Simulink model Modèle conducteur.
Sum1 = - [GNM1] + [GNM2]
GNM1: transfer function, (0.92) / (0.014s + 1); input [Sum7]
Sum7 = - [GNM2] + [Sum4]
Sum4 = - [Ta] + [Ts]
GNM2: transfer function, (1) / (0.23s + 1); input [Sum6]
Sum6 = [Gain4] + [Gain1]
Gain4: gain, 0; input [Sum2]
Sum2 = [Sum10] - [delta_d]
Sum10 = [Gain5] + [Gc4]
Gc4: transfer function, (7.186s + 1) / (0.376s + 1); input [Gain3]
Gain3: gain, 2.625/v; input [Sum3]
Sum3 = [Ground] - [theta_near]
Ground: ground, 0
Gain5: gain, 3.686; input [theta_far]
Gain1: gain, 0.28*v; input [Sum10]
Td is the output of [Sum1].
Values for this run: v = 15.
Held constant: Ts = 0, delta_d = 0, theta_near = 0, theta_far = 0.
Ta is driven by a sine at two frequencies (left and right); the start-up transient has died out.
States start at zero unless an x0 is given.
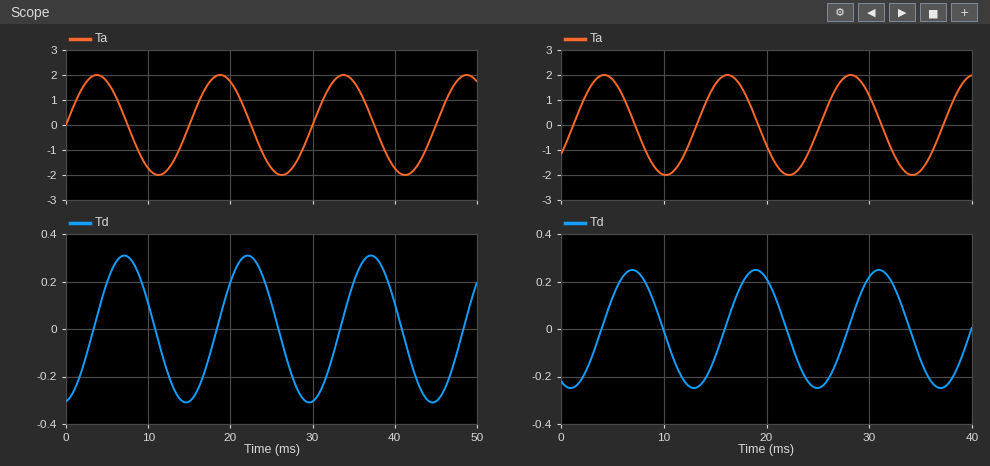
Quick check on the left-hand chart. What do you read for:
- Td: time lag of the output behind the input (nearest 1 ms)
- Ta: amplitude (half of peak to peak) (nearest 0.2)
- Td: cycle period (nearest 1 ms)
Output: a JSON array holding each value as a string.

["3 ms", "2.0", "15 ms"]
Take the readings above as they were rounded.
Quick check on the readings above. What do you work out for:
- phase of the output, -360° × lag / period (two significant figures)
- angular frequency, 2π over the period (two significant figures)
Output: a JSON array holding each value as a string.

["-72°", "0.42 rad/ms"]
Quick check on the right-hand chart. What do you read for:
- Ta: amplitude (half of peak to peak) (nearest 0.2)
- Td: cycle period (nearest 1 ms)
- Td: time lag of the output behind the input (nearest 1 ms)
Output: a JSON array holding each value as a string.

["2.0", "12 ms", "3 ms"]
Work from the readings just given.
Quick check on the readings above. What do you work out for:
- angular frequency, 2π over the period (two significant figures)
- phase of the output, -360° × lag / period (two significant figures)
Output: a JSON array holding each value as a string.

["0.52 rad/ms", "-90°"]
